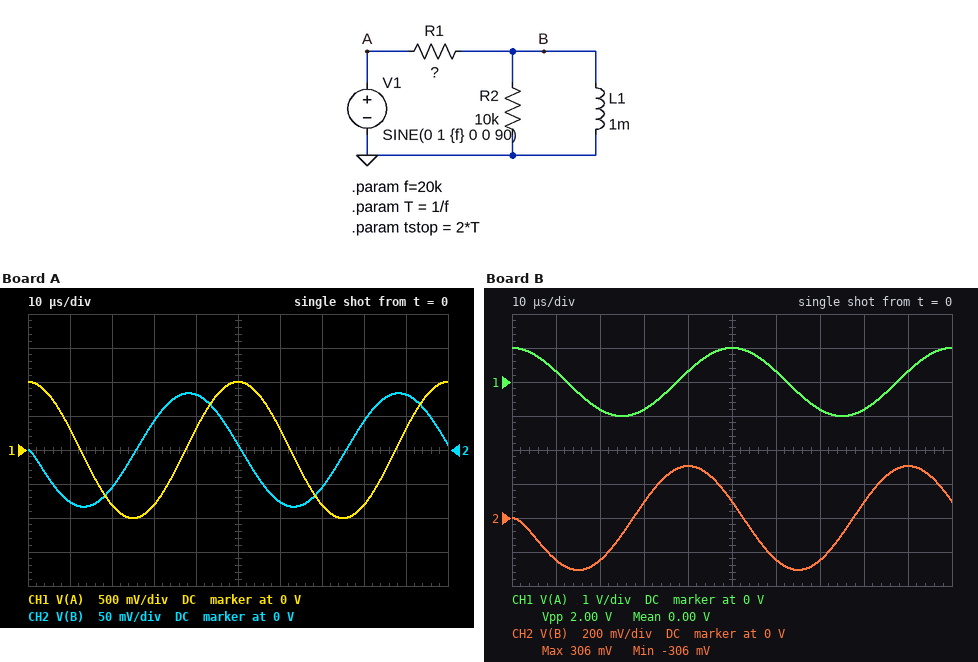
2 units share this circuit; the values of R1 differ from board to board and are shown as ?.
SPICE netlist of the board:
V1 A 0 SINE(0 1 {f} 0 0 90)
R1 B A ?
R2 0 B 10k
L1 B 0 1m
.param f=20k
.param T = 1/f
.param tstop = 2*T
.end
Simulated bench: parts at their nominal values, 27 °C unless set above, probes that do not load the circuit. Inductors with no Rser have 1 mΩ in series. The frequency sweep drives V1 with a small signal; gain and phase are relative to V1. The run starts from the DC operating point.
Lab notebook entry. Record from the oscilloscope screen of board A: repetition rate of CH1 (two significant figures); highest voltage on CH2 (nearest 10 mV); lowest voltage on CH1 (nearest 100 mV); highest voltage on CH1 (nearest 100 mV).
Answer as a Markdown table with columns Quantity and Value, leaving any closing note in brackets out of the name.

| Quantity | Value |
|---|---|
| repetition rate of CH1 | 20 kHz |
| highest voltage on CH2 | 80 mV |
| lowest voltage on CH1 | -1.0 V |
| highest voltage on CH1 | 1.0 V |
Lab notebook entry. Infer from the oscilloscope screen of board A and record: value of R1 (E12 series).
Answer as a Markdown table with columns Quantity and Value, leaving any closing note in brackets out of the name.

| Quantity | Value |
|---|---|
| value of R1 | 1.5 kΩ |
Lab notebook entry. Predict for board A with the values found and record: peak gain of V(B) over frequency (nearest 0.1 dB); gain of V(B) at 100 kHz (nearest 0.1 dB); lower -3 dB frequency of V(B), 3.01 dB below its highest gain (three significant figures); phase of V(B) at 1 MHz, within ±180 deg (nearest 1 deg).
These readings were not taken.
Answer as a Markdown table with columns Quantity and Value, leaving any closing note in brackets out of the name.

| Quantity | Value |
|---|---|
| peak gain of V(B) over frequency | -1.2 dB |
| gain of V(B) at 100 kHz | -8.5 dB |
| lower -3 dB frequency of V(B), 3.01 dB below its highest gain | 208 kHz |
| phase of V(B) at 1 MHz, within ±180 deg | 12 deg |
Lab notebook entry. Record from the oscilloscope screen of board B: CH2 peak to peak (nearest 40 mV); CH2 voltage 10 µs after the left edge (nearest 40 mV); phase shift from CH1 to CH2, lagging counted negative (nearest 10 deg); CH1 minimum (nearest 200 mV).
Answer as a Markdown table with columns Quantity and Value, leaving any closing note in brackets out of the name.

| Quantity | Value |
|---|---|
| CH2 peak to peak | 600 mV |
| CH2 voltage 10 µs after the left edge | -240 mV |
| phase shift from CH1 to CH2, lagging counted negative | 70 deg |
| CH1 minimum | -1.0 V |
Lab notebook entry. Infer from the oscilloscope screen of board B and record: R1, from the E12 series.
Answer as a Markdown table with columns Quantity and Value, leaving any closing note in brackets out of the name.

| Quantity | Value |
|---|---|
| R1, from the E12 series | 390 Ω |
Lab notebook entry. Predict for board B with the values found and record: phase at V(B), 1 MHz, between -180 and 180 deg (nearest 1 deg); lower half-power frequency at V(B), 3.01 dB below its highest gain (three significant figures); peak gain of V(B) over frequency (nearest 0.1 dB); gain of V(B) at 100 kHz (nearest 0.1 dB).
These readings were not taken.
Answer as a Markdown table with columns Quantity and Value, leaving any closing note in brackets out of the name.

| Quantity | Value |
|---|---|
| phase at V(B), 1 MHz, between -180 and 180 deg | 3 deg |
| lower half-power frequency at V(B), 3.01 dB below its highest gain | 59.7 kHz |
| peak gain of V(B) over frequency | -0.3 dB |
| gain of V(B) at 100 kHz | -1.7 dB |
